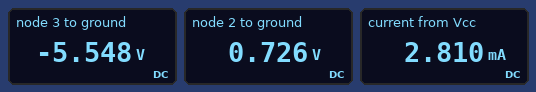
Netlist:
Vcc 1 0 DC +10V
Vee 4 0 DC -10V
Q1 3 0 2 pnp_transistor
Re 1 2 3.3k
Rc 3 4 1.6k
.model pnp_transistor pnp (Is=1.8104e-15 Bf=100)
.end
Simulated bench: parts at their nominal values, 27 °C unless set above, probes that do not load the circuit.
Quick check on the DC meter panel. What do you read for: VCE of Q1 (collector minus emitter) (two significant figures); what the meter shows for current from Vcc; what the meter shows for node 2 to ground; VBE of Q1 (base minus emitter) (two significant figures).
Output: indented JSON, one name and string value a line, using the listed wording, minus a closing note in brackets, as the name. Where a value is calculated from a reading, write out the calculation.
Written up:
{
  "VCE of Q1 (collector minus emitter)": "-5.548 V - 726 mV = -6.3 V",
  "what the meter shows for current from Vcc": "2.810 mA",
  "what the meter shows for node 2 to ground": "0.726 V",
  "VBE of Q1 (base minus emitter)": "0 V - 726 mV = -730 mV"
}
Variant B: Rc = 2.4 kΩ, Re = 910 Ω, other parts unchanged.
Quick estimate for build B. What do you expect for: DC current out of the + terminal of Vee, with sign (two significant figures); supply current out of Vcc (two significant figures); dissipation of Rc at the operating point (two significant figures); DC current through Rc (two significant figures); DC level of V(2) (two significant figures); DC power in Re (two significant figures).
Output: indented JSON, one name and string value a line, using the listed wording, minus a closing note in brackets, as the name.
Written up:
{
  "DC current out of the + terminal of Vee, with sign": "-4.5 mA",
  "supply current out of Vcc": "10 mA",
  "dissipation of Rc at the operating point": "48 mW",
  "DC current through Rc": "4.5 mA",
  "DC level of V(2)": "770 mV",
  "DC power in Re": "94 mW"
}
